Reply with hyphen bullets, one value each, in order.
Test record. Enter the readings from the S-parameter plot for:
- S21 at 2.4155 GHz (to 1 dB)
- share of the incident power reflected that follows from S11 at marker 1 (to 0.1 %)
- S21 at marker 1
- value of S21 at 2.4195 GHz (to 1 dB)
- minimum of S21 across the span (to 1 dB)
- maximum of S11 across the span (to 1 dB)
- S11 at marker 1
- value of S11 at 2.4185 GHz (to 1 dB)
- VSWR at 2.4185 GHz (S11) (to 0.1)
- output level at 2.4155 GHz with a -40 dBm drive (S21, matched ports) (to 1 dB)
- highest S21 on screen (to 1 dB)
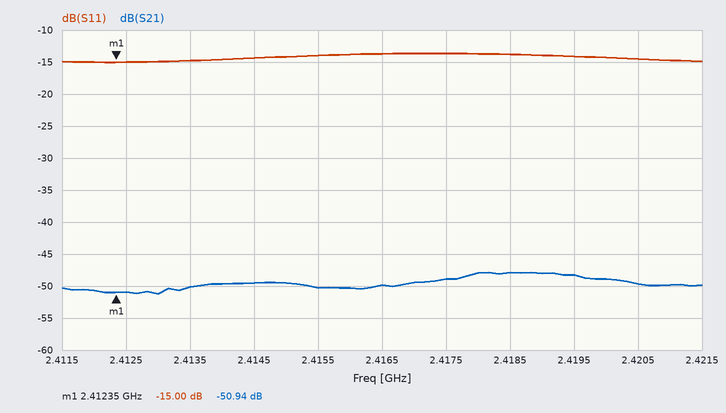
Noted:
- -50 dB
- 3.2 %
- -50.94 dB
- -48 dB
- -51 dB
- -14 dB
- -15.00 dB
- -14 dB
- 1.5
- -90 dBm
- -48 dB
